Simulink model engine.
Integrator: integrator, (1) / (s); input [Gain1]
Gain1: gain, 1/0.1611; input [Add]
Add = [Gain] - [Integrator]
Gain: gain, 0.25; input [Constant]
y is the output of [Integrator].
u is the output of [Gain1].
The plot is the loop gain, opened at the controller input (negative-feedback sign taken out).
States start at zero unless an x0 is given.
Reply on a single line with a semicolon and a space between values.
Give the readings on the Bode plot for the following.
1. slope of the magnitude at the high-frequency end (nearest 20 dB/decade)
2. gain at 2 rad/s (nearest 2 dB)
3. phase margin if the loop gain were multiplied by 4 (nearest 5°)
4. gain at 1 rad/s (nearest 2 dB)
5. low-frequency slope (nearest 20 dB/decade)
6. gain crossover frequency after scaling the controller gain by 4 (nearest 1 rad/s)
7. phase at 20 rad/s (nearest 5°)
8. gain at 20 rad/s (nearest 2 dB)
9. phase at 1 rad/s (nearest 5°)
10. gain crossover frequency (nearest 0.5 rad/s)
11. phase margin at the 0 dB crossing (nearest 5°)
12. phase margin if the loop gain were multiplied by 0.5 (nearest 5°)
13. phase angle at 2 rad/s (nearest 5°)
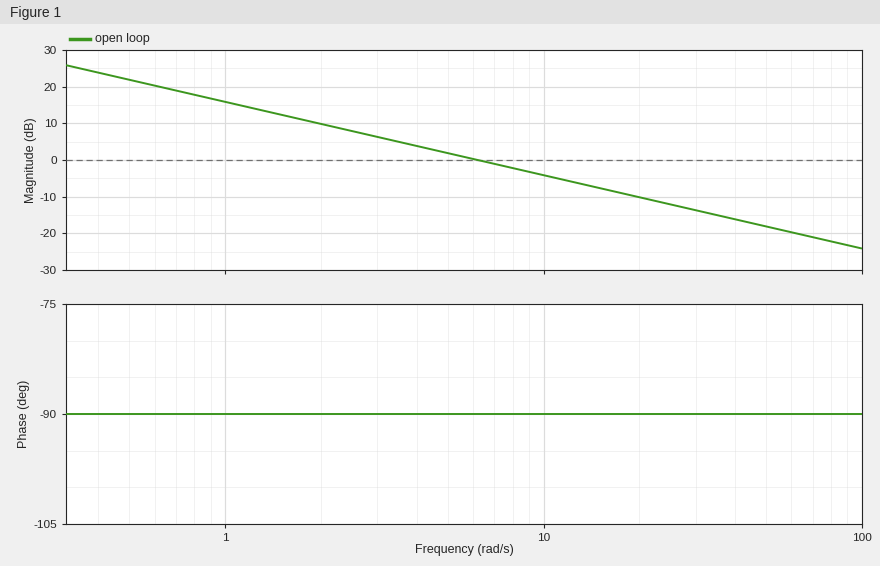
-20 dB/decade; 10 dB; 90°; 16 dB; -20 dB/decade; 25 rad/s; -90°; -10 dB; -90°; 6.0 rad/s; 90°; 90°; -90°
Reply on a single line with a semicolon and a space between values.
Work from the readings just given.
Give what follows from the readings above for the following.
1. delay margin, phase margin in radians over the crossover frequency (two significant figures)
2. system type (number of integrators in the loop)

0.26 s; 1
